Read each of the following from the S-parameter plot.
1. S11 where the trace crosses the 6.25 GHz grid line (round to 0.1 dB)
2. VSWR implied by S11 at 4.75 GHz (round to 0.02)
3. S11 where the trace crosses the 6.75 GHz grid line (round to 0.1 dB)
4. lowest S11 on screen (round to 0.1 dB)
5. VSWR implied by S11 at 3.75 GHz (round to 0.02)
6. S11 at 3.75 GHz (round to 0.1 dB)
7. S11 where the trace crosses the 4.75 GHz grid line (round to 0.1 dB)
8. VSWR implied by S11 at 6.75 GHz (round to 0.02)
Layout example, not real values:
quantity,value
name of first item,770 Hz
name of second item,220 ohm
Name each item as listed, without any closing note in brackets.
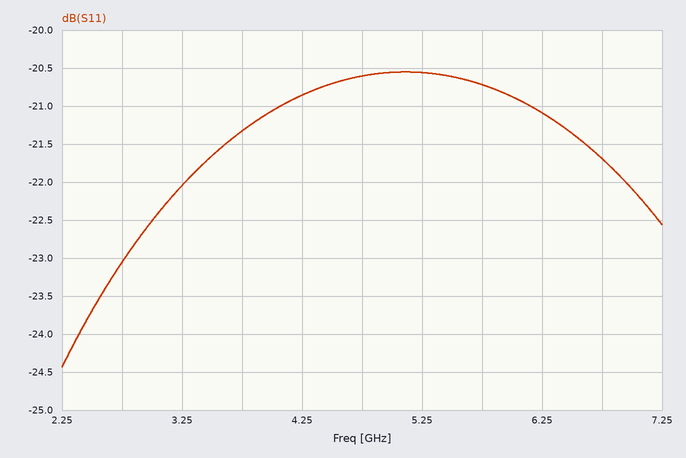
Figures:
quantity,value
S11 where the trace crosses the 6.25 GHz grid line,-21.1 dB
VSWR implied by S11 at 4.75 GHz,1.20
S11 where the trace crosses the 6.75 GHz grid line,-21.7 dB
lowest S11 on screen,-24.4 dB
VSWR implied by S11 at 3.75 GHz,1.18
S11 at 3.75 GHz,-21.3 dB
S11 where the trace crosses the 4.75 GHz grid line,-20.6 dB
VSWR implied by S11 at 6.75 GHz,1.18
